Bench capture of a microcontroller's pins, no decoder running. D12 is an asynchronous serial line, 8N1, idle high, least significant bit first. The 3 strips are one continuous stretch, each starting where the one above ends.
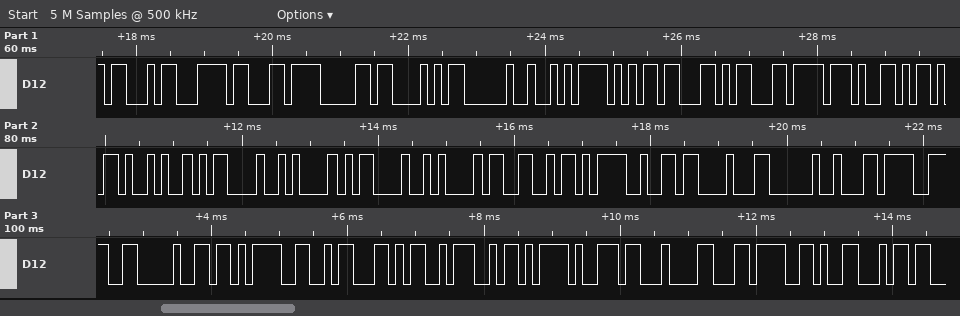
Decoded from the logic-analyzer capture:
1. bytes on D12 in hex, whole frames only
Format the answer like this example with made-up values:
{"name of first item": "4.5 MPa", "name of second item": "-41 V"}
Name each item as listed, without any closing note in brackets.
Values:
{"bytes on D12 in hex, whole frames only": "0xA3 0xBC 0xEC 0xB0 0xA8 0x20 0xEA 0xB5 0xAC 0xEC 0x97 0xAD 0x29 0x0D 0x0A 0x0D 0x0A 0x33 0xEB 0xB2 0x88 0x20 0xEC 0x9E 0x90 0xEB 0xA6 0xAC 0x3A 0xEB 0xB9 0x84 0xEC 0x96 0xB4"}
